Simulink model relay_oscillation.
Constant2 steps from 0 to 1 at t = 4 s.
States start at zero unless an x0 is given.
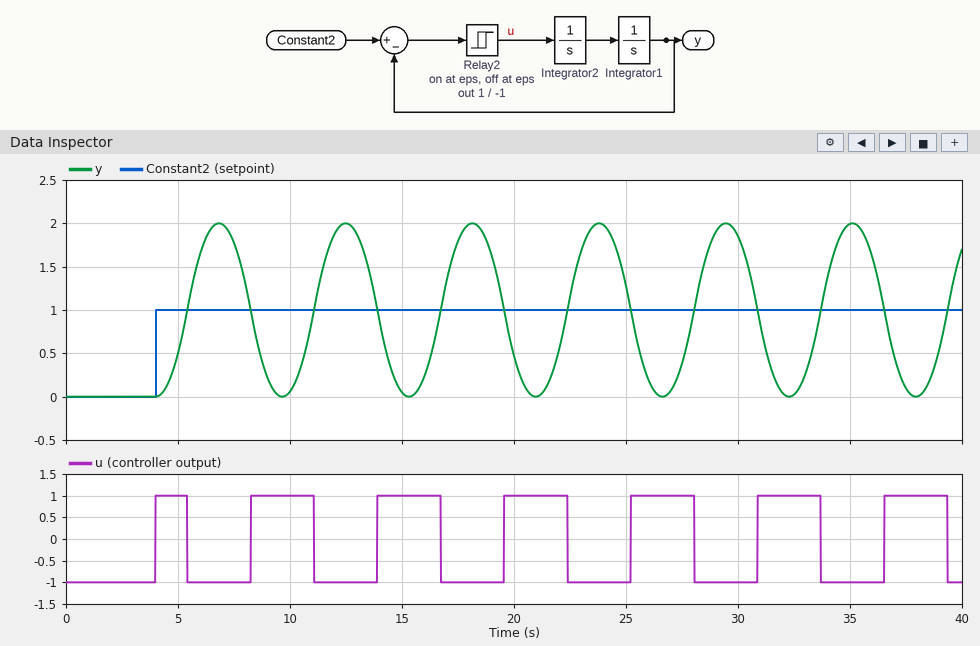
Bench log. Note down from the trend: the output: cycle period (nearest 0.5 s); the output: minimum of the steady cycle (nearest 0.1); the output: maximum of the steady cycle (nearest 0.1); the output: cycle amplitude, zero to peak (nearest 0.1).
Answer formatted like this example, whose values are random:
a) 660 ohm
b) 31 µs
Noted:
a) 5.5 s
b) 0.0
c) 2.0
d) 1.0
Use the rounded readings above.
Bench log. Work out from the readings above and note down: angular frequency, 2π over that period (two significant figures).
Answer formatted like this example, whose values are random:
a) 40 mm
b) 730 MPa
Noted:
a) 1.1 rad/s
